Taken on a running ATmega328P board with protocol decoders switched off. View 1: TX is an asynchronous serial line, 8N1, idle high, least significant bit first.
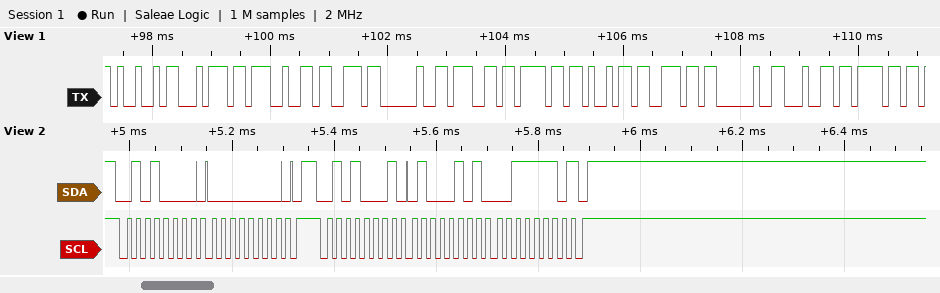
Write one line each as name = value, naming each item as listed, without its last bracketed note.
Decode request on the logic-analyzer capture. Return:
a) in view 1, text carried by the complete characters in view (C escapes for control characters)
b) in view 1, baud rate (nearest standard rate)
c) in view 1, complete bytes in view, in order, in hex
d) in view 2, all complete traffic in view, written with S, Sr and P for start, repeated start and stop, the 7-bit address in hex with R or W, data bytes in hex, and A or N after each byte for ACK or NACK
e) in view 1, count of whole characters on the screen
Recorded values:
in view 1, text carried by the complete characters in view = "It's goin do"
in view 1, baud rate = 9600 baud
in view 1, complete bytes in view, in order, in hex = 49 74 27 73 20 67 6F 69 6E 20 64 6F
in view 2, all complete traffic in view, written with S, Sr and P for start, repeated start and stop, the 7-bit address in hex with R or W, data bytes in hex, and A or N after each byte for ACK or NACK = S 28W A 00 A P S 28R A 45 A 3E N P
in view 1, count of whole characters on the screen = 12
